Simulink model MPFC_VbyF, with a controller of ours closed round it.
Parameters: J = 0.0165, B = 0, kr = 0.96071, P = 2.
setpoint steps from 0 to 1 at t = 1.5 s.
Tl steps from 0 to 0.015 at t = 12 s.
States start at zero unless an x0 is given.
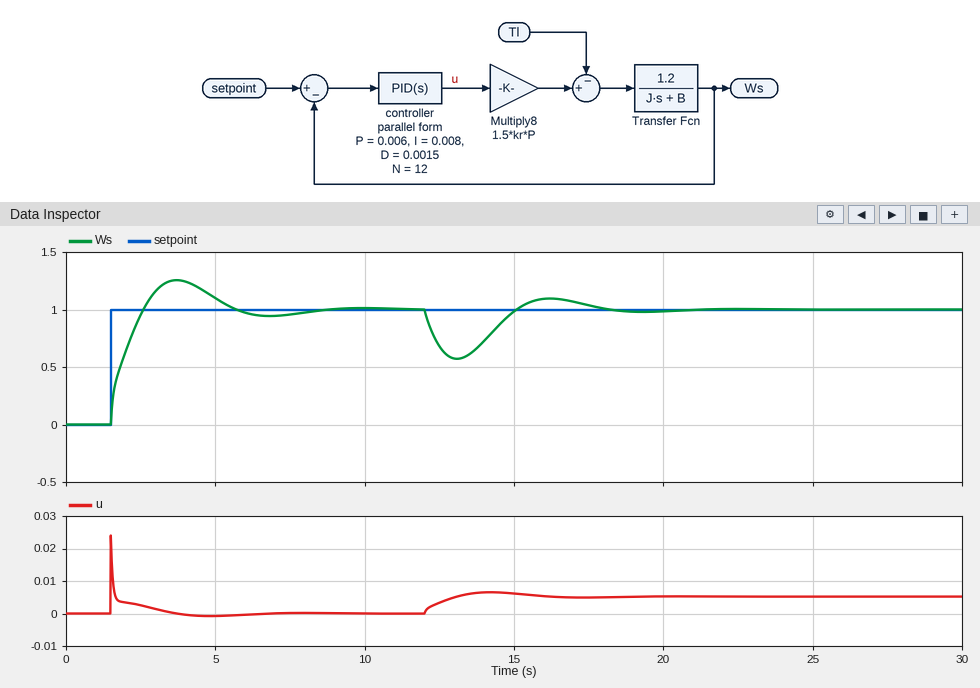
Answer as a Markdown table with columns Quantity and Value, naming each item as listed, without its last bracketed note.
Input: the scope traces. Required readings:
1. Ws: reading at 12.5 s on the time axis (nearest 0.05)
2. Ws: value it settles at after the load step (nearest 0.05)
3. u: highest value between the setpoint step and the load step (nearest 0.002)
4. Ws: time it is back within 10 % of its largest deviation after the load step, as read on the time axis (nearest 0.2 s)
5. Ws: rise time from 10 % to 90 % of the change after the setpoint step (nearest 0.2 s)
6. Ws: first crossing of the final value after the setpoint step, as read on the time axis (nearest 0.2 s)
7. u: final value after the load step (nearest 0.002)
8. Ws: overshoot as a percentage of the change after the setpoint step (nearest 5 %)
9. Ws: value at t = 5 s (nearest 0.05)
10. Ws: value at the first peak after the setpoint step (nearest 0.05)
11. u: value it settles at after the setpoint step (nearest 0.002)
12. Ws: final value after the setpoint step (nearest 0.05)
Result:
| Quantity | Value |
|---|---|
| Ws: reading at 12.5 s on the time axis | 0.70 |
| Ws: value it settles at after the load step | 1.00 |
| u: highest value between the setpoint step and the load step | 0.024 |
| Ws: time it is back within 10 % of its largest deviation after the load step, as read on the time axis | 17.4 s |
| Ws: rise time from 10 % to 90 % of the change after the setpoint step | 0.8 s |
| Ws: first crossing of the final value after the setpoint step, as read on the time axis | 2.6 s |
| u: final value after the load step | 0.006 |
| Ws: overshoot as a percentage of the change after the setpoint step | 25 % |
| Ws: value at t = 5 s | 1.10 |
| Ws: value at the first peak after the setpoint step | 1.25 |
| u: value it settles at after the setpoint step | 0.000 |
| Ws: final value after the setpoint step | 1.00 |
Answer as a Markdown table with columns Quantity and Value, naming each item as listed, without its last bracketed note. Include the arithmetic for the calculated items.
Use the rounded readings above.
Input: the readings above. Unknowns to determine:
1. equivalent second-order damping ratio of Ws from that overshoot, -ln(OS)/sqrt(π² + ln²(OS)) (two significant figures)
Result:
| Quantity | Value |
|---|---|
| equivalent second-order damping ratio of Ws from that overshoot, -ln(OS)/sqrt(π² + ln²(OS)) | ln(0.25) = -1.386; 1.386 / sqrt(9.870 + 1.922) = 0.40 |
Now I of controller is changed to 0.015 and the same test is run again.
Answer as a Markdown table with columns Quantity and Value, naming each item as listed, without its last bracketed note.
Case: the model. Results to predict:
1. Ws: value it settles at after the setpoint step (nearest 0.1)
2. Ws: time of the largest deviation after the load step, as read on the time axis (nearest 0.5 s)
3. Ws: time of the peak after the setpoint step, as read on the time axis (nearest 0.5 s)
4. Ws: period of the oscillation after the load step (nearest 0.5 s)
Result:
| Quantity | Value |
|---|---|
| Ws: value it settles at after the setpoint step | 1.0 |
| Ws: time of the largest deviation after the load step, as read on the time axis | 13.0 s |
| Ws: time of the peak after the setpoint step, as read on the time axis | 3.0 s |
| Ws: period of the oscillation after the load step | 4.5 s |
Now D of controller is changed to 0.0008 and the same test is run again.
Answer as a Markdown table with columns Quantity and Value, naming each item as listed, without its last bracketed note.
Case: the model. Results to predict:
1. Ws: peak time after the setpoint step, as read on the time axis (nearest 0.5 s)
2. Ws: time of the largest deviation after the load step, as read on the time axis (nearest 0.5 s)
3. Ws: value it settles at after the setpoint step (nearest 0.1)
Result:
| Quantity | Value |
|---|---|
| Ws: peak time after the setpoint step, as read on the time axis | 3.5 s |
| Ws: time of the largest deviation after the load step, as read on the time axis | 13.0 s |
| Ws: value it settles at after the setpoint step | 1.0 |
